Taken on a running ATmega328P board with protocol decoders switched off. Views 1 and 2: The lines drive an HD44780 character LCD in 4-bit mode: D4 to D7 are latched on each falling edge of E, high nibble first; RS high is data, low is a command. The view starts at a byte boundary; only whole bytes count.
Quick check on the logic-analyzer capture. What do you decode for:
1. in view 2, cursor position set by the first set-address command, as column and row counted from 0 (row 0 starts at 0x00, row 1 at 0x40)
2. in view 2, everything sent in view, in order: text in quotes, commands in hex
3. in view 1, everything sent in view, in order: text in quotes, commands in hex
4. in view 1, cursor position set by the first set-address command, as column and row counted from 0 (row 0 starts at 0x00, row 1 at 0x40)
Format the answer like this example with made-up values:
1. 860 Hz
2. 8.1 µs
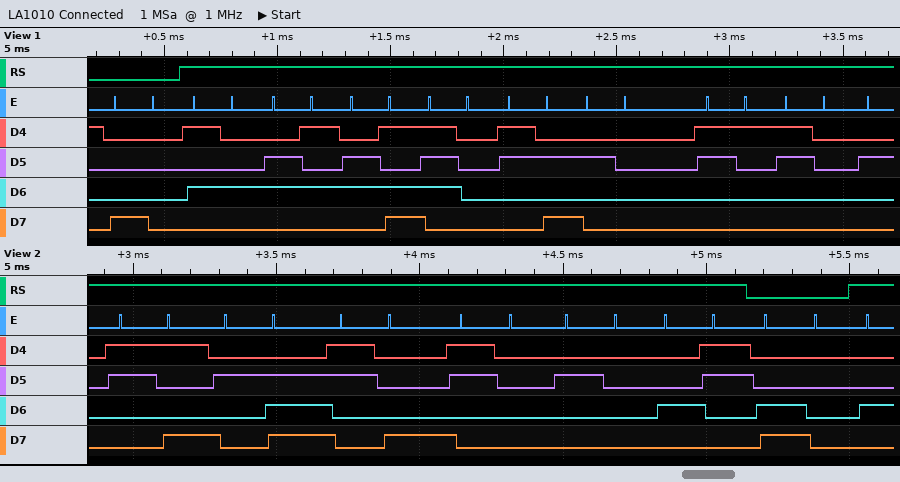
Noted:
1. column 0, row 1
2. "9.80 C" 0xC0
3. 0x80 "Temp: 10"
4. column 0, row 0
